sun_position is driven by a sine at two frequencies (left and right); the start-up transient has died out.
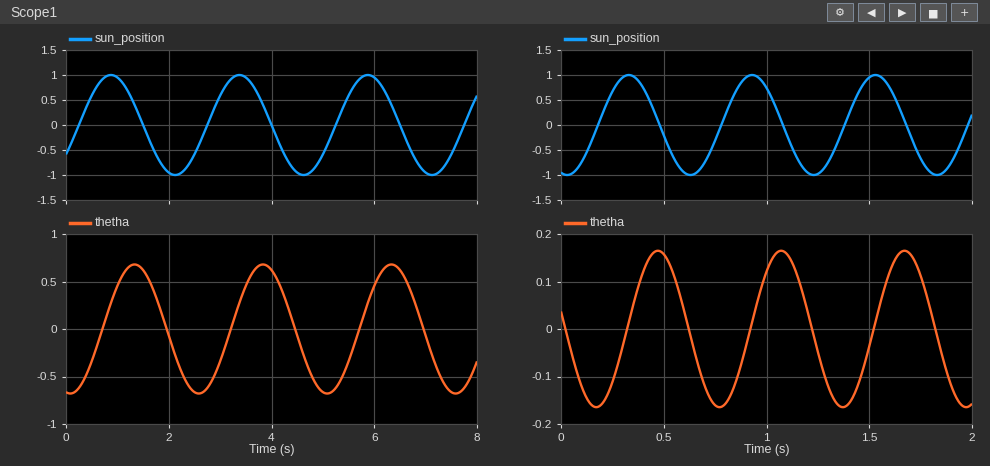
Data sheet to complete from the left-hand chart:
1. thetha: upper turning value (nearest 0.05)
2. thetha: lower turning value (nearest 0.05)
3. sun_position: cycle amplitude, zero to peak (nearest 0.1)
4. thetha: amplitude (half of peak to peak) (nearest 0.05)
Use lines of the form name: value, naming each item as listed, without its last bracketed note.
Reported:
thetha: upper turning value: 0.70
thetha: lower turning value: -0.70
sun_position: cycle amplitude, zero to peak: 1.0
thetha: amplitude (half of peak to peak): 0.70
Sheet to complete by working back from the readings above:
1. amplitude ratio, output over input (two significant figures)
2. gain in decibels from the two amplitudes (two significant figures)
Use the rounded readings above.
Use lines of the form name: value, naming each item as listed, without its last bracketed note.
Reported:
amplitude ratio, output over input: 0.70
gain in decibels from the two amplitudes: -3.1 dB
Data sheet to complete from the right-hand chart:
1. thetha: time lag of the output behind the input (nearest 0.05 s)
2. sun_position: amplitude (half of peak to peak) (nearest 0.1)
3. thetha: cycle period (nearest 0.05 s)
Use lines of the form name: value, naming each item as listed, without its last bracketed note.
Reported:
thetha: time lag of the output behind the input: 0.15 s
sun_position: amplitude (half of peak to peak): 1.0
thetha: cycle period: 0.60 s
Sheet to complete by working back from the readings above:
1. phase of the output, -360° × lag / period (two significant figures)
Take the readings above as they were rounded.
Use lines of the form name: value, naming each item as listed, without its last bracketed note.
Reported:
phase of the output, -360° × lag / period: -90°
